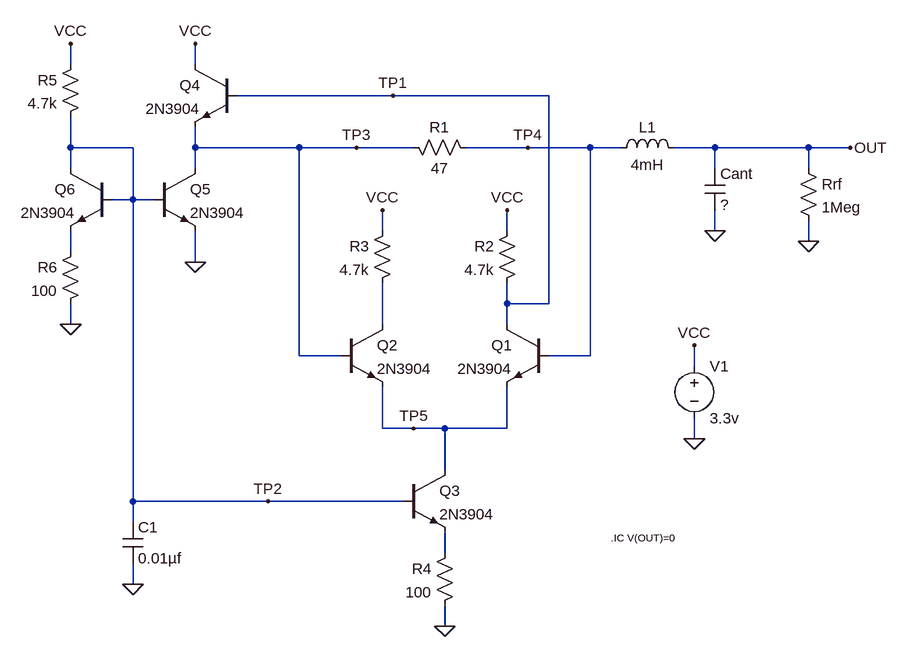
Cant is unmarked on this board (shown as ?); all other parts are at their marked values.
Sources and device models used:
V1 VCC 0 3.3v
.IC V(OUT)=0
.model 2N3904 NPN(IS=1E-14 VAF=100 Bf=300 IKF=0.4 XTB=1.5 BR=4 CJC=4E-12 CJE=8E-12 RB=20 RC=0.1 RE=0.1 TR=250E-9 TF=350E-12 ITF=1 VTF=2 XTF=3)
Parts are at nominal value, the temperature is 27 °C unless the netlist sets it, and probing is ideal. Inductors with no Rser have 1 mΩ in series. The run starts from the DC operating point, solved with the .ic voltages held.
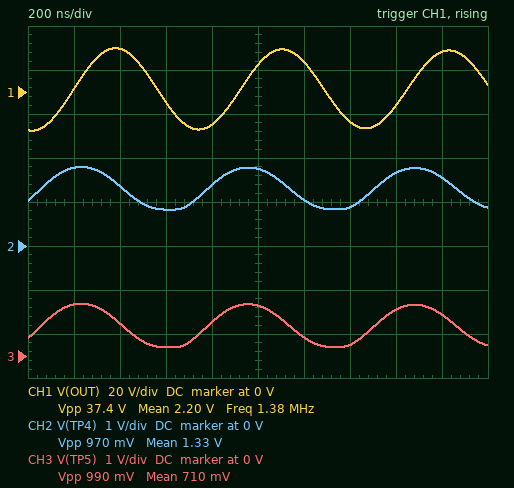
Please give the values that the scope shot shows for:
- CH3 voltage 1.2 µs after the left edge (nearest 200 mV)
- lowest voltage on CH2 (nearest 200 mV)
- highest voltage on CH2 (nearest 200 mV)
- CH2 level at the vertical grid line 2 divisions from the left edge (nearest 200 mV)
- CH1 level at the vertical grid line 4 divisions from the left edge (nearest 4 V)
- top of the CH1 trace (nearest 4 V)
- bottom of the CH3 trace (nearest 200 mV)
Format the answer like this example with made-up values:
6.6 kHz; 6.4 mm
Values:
400 mV; 800 mV; 1.8 V; 1.4 V; -16 V; 20 V; 200 mV
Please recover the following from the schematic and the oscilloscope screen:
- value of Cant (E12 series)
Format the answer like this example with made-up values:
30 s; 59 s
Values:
3.3 pF
